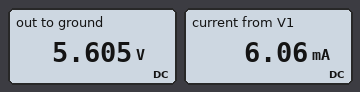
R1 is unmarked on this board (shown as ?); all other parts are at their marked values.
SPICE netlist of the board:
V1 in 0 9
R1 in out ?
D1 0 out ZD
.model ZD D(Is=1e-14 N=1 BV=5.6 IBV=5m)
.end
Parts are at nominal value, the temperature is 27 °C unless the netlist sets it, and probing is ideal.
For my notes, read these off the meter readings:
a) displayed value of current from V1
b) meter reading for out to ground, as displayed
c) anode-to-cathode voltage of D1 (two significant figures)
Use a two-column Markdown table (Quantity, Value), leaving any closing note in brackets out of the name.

| Quantity | Value |
|---|---|
| displayed value of current from V1 | 6.06 mA |
| meter reading for out to ground, as displayed | 5.605 V |
| anode-to-cathode voltage of D1 | -5.6 V |
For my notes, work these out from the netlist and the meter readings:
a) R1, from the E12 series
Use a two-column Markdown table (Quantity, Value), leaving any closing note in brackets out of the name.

| Quantity | Value |
|---|---|
| R1, from the E12 series | 560 Ω |
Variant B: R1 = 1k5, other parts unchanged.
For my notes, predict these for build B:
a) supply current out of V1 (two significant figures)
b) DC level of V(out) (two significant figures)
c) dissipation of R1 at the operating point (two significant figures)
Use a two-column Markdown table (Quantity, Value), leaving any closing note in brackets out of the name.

| Quantity | Value |
|---|---|
| supply current out of V1 | 2.3 mA |
| DC level of V(out) | 5.6 V |
| dissipation of R1 at the operating point | 7.8 mW |
